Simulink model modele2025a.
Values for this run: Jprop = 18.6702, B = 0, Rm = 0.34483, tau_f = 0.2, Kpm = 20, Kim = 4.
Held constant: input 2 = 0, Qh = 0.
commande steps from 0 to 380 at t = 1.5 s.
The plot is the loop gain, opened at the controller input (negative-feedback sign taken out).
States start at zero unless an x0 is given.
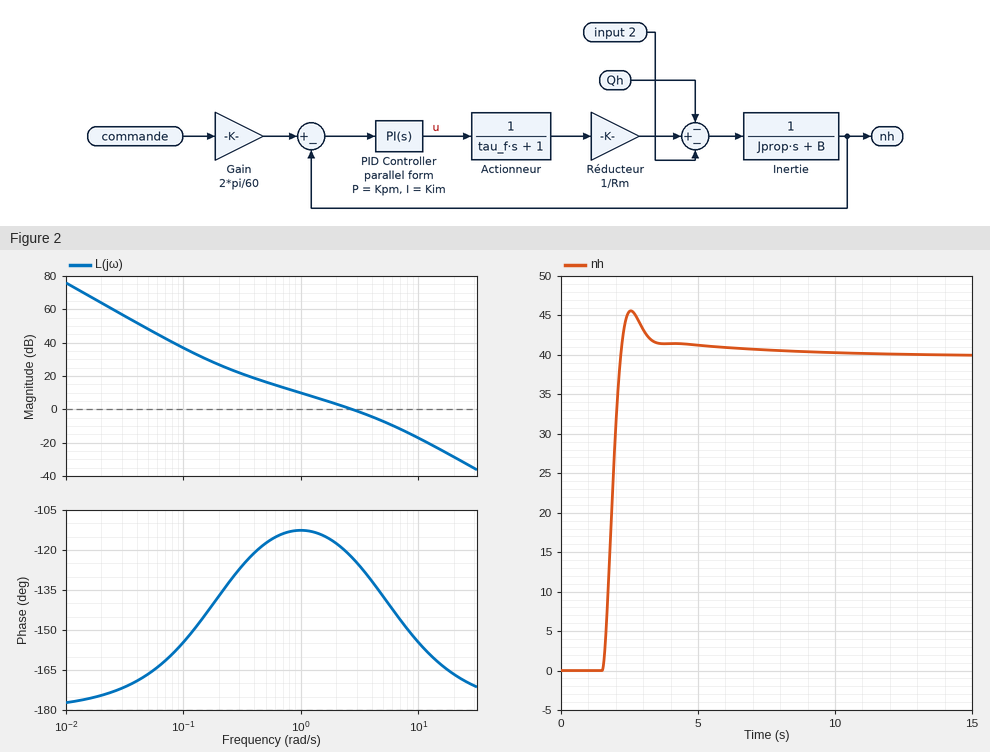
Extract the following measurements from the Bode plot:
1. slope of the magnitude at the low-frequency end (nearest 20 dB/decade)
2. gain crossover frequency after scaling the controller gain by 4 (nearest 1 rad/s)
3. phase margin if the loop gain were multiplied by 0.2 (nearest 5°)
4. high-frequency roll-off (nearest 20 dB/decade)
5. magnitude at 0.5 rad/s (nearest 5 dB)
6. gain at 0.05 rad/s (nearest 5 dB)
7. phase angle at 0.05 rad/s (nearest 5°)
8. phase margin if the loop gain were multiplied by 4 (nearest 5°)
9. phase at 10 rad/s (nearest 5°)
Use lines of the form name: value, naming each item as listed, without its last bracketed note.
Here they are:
slope of the magnitude at the low-frequency end: -40 dB/decade
gain crossover frequency after scaling the controller gain by 4: 7 rad/s
phase margin if the loop gain were multiplied by 0.2: 65°
high-frequency roll-off: -40 dB/decade
magnitude at 0.5 rad/s: 15 dB
gain at 0.05 rad/s: 50 dB
phase angle at 0.05 rad/s: -165°
phase margin if the loop gain were multiplied by 4: 35°
phase at 10 rad/s: -155°
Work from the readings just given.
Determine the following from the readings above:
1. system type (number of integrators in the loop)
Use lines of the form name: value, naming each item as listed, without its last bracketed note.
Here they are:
system type: 2
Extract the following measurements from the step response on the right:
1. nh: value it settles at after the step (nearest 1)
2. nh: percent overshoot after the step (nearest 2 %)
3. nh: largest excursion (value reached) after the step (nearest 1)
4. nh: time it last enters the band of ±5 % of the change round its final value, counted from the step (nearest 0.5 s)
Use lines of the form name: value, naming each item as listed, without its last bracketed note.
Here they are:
nh: value it settles at after the step: 40
nh: percent overshoot after the step: 14 %
nh: largest excursion (value reached) after the step: 46
nh: time it last enters the band of ±5 % of the change round its final value, counted from the step: 2.0 s
